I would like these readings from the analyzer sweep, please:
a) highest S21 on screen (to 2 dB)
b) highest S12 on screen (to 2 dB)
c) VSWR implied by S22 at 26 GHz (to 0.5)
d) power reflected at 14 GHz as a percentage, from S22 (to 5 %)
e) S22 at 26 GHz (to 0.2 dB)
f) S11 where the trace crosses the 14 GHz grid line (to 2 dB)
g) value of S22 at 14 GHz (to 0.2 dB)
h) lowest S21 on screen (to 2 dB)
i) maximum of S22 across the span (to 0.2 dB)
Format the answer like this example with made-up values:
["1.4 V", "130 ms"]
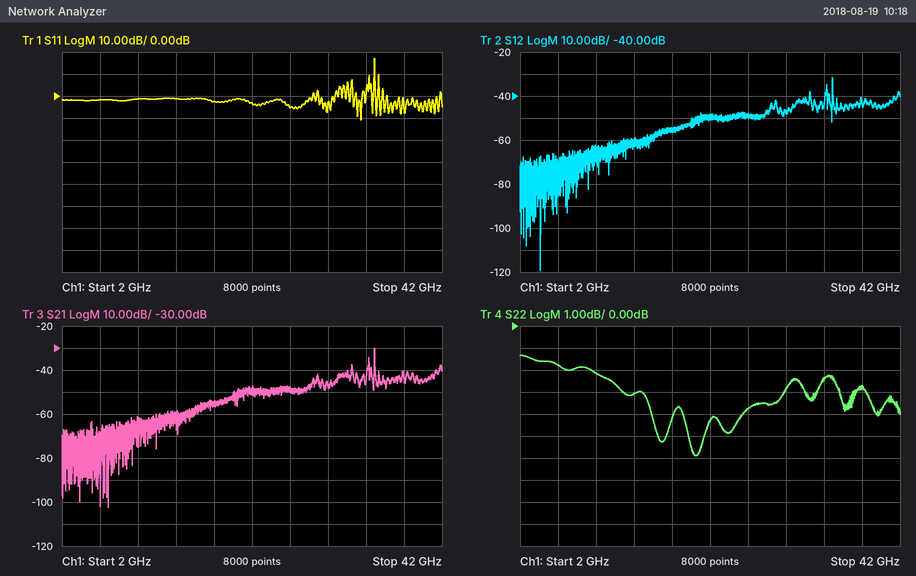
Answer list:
["-30 dB", "-32 dB", "4.5", "50 %", "-3.8 dB", "-2 dB", "-3.0 dB", "-102 dB", "-1.4 dB"]
